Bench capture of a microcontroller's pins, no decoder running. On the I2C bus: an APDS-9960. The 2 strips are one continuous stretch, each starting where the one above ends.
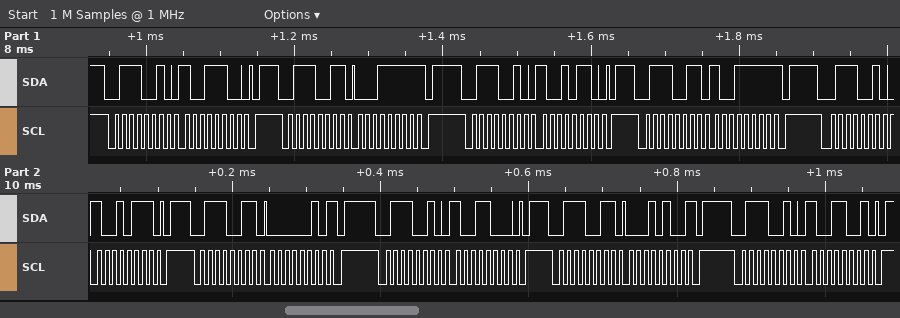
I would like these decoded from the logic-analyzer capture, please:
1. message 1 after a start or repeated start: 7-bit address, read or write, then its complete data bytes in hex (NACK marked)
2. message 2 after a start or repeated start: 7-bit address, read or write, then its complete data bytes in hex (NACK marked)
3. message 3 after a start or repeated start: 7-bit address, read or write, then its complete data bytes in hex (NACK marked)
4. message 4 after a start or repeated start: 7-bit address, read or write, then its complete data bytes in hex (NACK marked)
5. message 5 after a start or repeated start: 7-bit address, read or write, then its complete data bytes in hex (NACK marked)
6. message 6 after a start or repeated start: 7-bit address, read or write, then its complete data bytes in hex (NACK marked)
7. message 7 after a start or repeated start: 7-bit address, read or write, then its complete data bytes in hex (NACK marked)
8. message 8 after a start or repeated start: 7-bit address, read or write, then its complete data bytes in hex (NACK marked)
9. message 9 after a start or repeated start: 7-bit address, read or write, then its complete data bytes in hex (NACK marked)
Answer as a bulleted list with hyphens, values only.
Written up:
- 0x39 write: 9C
- 0x39 read: 1F NACK
- 0x39 write: 96
- 0x39 read: 9F NACK
- 0x39 write: 97
- 0x39 read: 02 NACK
- 0x39 write: 98
- 0x39 read: 14 NACK
- 0x39 write: 99
